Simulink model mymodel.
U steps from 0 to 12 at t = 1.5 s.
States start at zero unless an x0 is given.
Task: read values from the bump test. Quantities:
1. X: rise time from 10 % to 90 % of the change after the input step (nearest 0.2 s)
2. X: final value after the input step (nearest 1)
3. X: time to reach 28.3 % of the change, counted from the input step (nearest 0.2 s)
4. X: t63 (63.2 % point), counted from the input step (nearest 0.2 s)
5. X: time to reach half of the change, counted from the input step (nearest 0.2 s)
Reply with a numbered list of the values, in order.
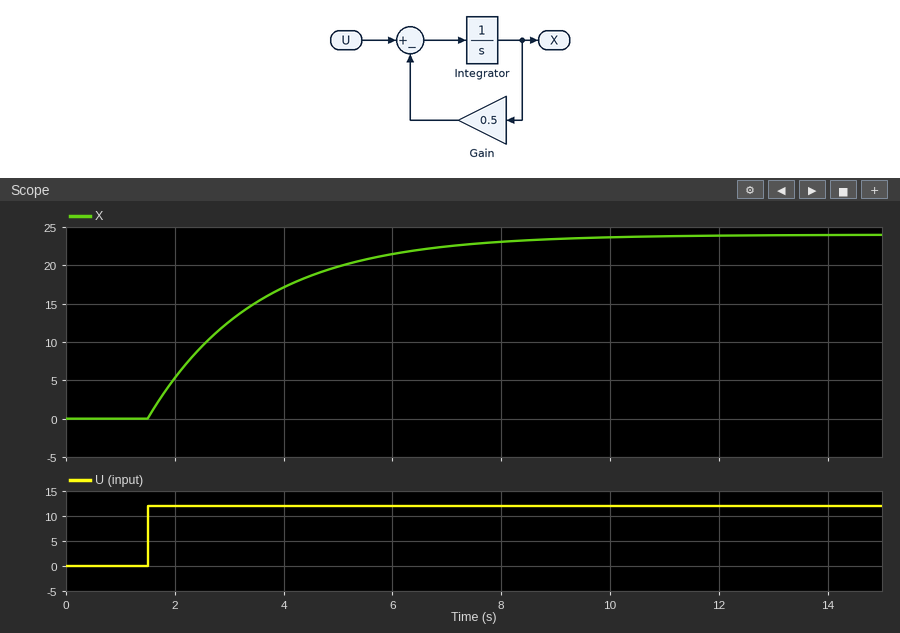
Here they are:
1. 4.4 s
2. 24
3. 0.6 s
4. 2.0 s
5. 1.4 s
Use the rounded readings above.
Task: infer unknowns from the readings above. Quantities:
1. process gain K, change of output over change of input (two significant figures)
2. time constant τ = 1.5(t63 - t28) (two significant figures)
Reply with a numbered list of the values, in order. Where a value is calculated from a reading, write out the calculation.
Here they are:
1. (24 - 0) / 12 = 2.0
2. 1.5 × (2 - 0.6) = 2.1 s
